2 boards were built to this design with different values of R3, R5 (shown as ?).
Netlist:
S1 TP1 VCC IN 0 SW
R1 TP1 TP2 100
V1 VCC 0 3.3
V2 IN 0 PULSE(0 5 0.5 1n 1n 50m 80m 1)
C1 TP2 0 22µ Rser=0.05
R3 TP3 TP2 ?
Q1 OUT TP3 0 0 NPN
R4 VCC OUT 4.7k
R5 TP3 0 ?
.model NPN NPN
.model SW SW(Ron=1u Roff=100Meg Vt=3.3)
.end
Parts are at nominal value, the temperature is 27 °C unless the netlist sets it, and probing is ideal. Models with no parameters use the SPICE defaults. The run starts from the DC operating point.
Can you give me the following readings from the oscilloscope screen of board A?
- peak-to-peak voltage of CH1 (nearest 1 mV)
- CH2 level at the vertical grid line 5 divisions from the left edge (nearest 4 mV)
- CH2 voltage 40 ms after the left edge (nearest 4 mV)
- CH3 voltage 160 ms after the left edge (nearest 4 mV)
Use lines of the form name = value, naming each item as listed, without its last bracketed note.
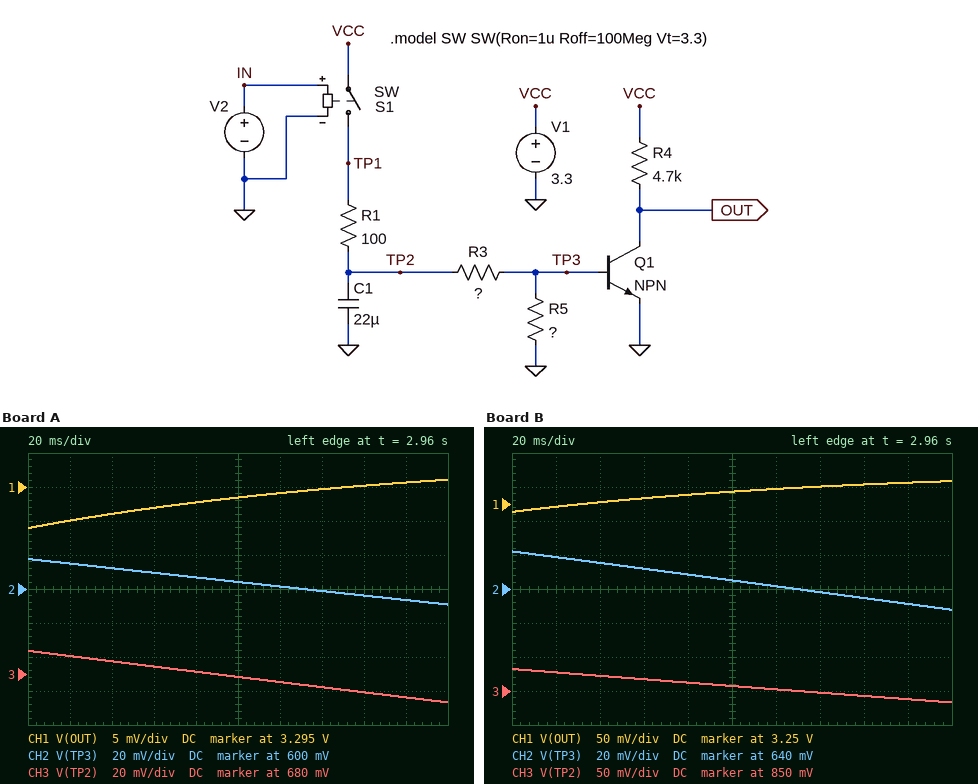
peak-to-peak voltage of CH1 = 7 mV
CH2 level at the vertical grid line 5 divisions from the left edge = 604 mV
CH2 voltage 40 ms after the left edge = 612 mV
CH3 voltage 160 ms after the left edge = 668 mV
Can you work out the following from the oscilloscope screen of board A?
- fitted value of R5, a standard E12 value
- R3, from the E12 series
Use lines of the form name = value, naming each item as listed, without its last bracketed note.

fitted value of R5, a standard E12 value = 180 kΩ
R3, from the E12 series = 22 kΩ
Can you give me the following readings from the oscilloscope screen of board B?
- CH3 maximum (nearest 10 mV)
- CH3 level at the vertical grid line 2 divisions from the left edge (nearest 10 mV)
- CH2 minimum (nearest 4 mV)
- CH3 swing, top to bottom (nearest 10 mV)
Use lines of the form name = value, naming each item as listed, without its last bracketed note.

CH3 maximum = 880 mV
CH3 level at the vertical grid line 2 divisions from the left edge = 870 mV
CH2 minimum = 628 mV
CH3 swing, top to bottom = 50 mV
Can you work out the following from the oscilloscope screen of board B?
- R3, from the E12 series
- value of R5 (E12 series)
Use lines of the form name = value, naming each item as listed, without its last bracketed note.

R3, from the E12 series = 39 kΩ
value of R5 = 120 kΩ
